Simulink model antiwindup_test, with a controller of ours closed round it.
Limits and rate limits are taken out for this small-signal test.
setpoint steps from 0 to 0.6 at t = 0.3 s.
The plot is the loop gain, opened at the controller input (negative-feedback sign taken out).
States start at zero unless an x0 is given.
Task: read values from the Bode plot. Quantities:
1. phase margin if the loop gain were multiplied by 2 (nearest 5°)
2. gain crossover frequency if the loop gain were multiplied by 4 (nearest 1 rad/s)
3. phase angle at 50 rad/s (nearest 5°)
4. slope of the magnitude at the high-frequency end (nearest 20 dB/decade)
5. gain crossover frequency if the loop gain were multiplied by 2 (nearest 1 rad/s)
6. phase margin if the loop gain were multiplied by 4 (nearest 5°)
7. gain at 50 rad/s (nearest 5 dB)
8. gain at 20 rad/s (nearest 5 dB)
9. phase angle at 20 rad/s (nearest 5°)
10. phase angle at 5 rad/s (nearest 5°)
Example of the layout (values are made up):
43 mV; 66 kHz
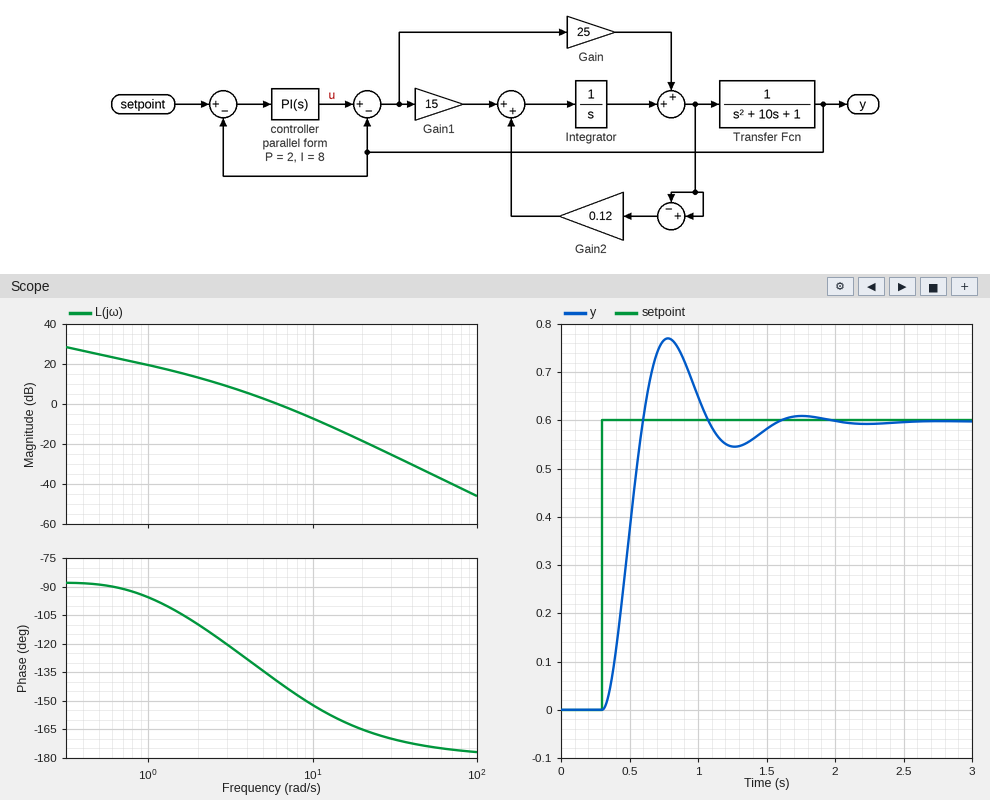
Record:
30°; 14 rad/s; -175°; -40 dB/decade; 9 rad/s; 20°; -35 dB; -20 dB; -165°; -135°
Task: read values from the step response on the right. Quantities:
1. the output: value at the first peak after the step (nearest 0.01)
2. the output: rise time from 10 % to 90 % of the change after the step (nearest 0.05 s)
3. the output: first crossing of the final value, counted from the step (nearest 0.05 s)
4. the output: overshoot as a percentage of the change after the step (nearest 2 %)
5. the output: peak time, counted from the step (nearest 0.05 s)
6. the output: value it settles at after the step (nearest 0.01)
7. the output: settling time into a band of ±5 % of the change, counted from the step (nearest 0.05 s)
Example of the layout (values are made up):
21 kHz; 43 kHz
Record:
0.77; 0.20 s; 0.30 s; 28 %; 0.50 s; 0.60; 1.15 s
